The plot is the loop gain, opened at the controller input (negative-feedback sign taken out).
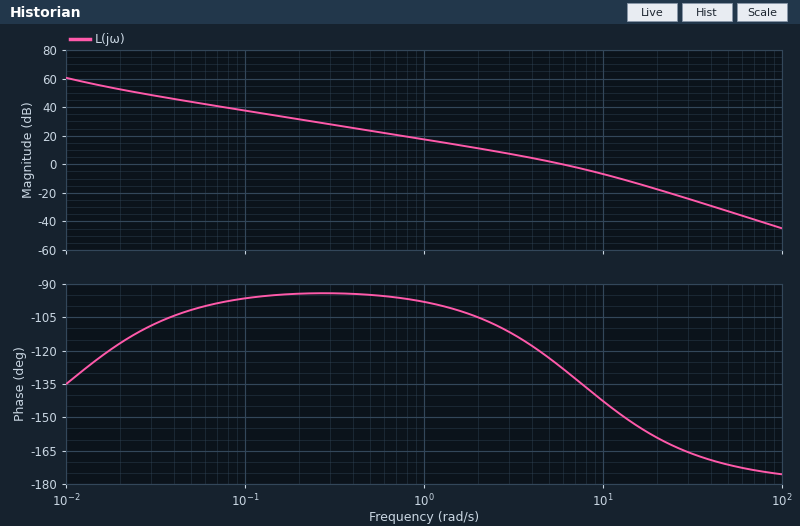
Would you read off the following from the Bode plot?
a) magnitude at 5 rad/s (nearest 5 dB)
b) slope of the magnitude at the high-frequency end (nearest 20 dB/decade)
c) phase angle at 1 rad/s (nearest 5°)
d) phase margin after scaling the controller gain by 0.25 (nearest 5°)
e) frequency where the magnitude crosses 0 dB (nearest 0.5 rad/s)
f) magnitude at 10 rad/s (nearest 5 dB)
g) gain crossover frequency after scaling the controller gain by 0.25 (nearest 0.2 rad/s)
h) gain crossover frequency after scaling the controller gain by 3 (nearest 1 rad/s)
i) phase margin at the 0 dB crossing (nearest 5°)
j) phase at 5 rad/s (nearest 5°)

0 dB
-40 dB/decade
-100°
75°
6.0 rad/s
-5 dB
1.8 rad/s
12 rad/s
50°
-125°
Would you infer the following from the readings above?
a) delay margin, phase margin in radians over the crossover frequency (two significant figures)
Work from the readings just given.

0.15 s
